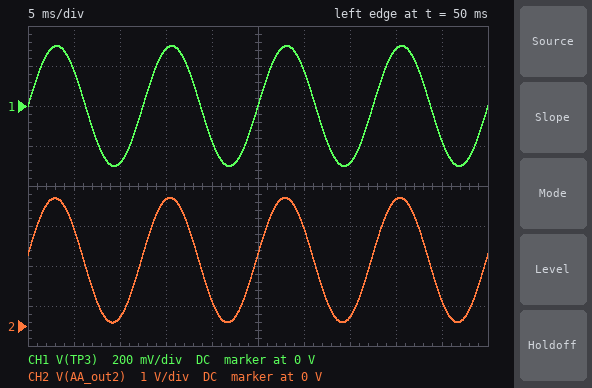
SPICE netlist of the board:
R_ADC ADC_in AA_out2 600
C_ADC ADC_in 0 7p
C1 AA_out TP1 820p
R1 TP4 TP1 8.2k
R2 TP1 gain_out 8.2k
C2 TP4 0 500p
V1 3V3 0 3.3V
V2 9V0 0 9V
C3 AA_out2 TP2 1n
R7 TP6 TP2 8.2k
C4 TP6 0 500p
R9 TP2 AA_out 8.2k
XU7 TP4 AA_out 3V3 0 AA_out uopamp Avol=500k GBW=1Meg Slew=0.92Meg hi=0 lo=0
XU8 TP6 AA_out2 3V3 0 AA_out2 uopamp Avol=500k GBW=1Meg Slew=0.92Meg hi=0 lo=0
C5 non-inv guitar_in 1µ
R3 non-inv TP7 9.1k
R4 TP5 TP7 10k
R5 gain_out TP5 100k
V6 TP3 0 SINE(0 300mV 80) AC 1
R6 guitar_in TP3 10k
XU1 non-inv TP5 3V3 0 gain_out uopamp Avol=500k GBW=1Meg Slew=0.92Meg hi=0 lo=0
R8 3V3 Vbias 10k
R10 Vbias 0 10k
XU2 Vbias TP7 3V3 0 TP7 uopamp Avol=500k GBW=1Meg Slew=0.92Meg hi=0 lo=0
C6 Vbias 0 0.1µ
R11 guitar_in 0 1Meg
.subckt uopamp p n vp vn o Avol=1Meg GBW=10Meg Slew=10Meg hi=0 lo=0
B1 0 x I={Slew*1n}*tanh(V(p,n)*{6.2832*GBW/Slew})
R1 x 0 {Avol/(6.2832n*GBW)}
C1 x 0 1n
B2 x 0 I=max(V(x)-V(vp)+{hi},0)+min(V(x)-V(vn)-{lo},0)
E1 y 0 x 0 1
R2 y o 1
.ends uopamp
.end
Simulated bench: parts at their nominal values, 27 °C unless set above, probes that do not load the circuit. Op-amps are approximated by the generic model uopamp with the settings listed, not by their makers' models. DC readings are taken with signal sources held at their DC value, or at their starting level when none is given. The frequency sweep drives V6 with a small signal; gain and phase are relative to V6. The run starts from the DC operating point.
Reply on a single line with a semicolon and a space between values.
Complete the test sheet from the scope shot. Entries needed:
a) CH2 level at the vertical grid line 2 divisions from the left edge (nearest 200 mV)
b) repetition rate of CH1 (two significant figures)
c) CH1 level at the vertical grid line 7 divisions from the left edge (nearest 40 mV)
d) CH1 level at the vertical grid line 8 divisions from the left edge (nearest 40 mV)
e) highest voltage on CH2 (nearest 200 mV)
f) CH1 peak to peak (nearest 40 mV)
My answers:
200 mV; 80 Hz; -280 mV; 280 mV; 3.2 V; 600 mV
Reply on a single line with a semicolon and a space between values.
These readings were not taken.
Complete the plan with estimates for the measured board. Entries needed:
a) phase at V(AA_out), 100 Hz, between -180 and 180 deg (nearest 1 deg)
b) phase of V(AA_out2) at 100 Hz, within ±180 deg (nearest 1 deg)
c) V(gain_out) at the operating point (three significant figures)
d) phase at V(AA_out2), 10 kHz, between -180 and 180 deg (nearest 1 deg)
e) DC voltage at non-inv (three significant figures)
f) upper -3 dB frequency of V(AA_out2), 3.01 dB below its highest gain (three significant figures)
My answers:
4 deg; 4 deg; 1.65 V; -68 deg; 1.65 V; 21.1 kHz
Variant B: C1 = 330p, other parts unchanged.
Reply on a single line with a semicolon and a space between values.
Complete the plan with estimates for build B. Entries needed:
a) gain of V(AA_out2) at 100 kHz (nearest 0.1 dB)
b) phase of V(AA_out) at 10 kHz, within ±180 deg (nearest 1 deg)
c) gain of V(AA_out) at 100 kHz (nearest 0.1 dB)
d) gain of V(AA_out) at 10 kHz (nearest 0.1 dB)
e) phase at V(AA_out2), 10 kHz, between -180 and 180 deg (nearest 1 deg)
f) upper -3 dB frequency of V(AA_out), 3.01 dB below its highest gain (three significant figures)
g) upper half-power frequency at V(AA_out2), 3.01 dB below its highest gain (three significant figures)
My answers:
-27.9 dB; -35 deg; -5.1 dB; 13.6 dB; -67 deg; 22.0 kHz; 18.5 kHz
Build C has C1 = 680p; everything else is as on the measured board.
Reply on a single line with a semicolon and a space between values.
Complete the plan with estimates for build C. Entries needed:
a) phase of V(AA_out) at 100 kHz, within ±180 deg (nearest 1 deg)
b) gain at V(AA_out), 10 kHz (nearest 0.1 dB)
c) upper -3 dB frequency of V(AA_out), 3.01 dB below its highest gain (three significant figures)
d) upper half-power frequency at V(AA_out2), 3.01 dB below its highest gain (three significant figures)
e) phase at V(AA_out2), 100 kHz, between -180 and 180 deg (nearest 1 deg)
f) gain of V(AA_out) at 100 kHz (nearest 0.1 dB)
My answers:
158 deg; 13.9 dB; 25.3 kHz; 20.4 kHz; -5 deg; -9.0 dB
